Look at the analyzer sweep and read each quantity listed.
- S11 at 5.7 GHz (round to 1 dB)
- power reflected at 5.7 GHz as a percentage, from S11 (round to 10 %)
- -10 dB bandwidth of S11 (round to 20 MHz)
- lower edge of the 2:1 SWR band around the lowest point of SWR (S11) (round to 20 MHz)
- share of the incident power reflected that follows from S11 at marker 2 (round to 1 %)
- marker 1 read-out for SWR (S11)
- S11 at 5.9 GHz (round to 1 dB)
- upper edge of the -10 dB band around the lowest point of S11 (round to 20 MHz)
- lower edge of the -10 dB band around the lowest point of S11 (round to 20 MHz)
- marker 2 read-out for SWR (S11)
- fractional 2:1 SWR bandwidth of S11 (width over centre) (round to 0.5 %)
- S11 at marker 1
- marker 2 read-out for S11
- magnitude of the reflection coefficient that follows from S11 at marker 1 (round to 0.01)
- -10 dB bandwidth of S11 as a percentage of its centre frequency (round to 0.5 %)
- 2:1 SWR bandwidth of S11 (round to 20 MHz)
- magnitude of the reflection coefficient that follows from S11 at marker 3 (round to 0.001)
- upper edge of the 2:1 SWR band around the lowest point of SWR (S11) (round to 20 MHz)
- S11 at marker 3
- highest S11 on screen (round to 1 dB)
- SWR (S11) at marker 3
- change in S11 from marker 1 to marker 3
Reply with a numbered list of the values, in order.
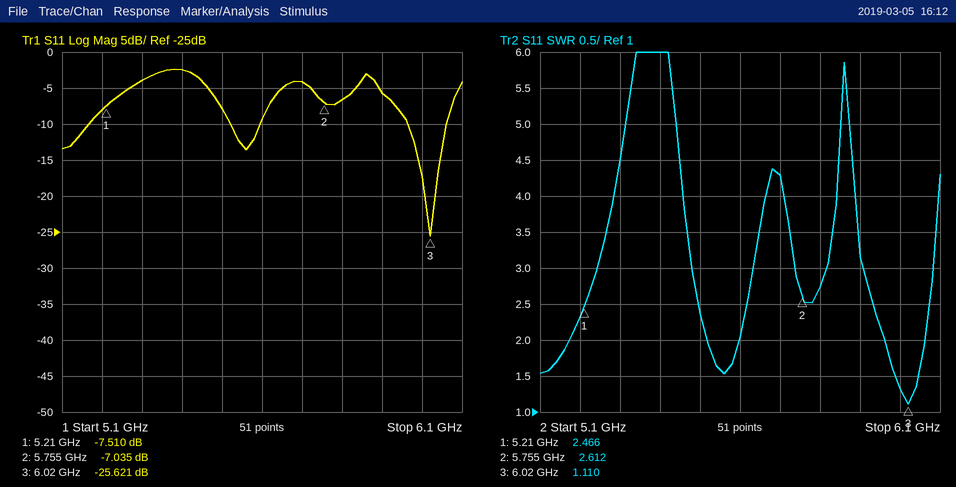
1. -4 dB
2. 40 %
3. 100 MHz
4. 5.96 GHz
5. 20 %
6. 2.466
7. -6 dB
8. 6.06 GHz
9. 5.96 GHz
10. 2.612
11. 1.5 %
12. -7.510 dB
13. -7.035 dB
14. 0.42
15. 1.5 %
16. 100 MHz
17. 0.052
18. 6.06 GHz
19. -25.621 dB
20. -2 dB
21. 1.110
22. -18.111 dB
